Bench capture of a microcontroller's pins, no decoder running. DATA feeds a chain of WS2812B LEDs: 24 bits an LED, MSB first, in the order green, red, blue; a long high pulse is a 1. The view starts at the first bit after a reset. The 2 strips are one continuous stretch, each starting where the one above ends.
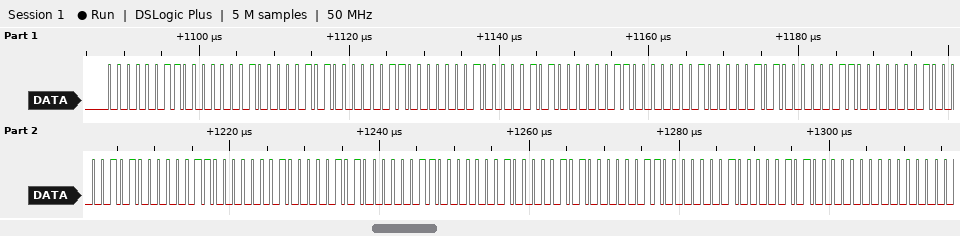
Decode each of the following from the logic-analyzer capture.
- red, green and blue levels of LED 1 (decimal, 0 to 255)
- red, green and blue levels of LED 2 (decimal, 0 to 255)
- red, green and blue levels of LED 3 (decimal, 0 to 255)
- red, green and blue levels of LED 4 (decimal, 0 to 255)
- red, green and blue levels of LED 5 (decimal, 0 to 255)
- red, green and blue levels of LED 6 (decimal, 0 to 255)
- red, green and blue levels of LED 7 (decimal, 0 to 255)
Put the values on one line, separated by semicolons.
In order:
1, 3, 5; 1, 3, 5; 1, 3, 5; 1, 3, 5; 1, 3, 5; 1, 3, 5; 1, 3, 5
